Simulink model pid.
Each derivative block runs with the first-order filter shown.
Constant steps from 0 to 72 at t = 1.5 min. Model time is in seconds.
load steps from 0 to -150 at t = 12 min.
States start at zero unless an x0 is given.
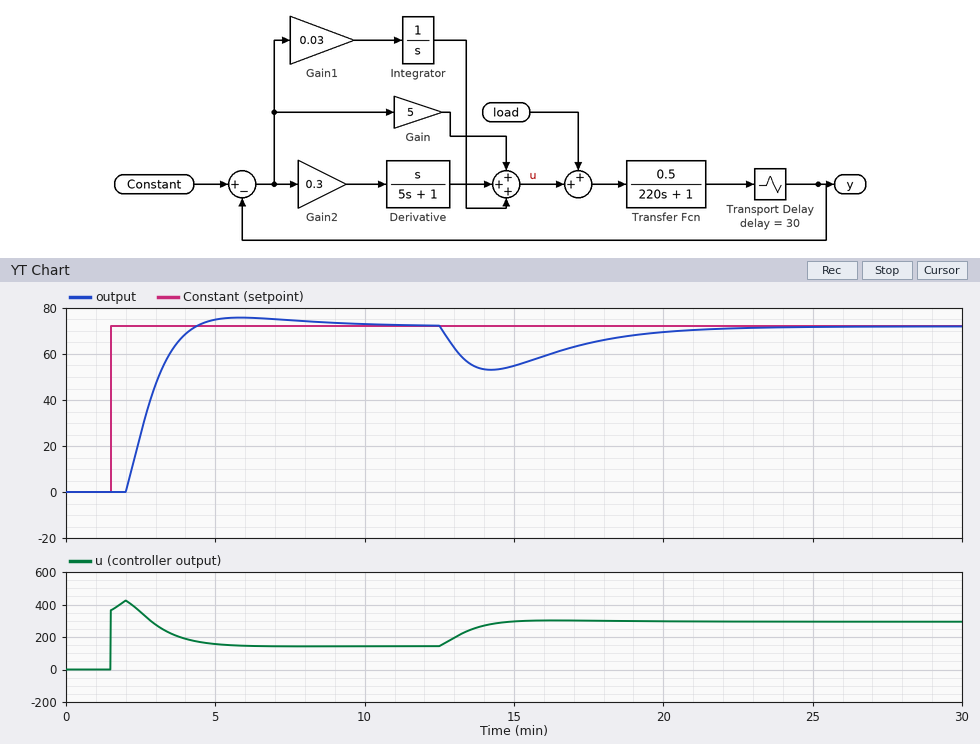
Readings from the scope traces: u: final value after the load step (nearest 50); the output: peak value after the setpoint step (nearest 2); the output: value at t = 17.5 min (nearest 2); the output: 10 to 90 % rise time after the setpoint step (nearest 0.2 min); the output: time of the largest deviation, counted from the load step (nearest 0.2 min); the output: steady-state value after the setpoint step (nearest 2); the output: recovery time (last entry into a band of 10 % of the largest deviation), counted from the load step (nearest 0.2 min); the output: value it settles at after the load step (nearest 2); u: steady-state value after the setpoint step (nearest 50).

300
76
64
1.6 min
2.2 min
72
8.6 min
72
150
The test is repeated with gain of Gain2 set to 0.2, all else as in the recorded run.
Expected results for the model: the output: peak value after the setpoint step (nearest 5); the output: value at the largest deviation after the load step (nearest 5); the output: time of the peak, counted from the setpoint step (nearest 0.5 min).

75
55
4.5 min
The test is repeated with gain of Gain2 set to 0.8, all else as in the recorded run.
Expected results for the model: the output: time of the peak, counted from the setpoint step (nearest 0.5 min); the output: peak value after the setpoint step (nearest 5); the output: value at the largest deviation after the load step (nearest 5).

4.5 min
75
55
